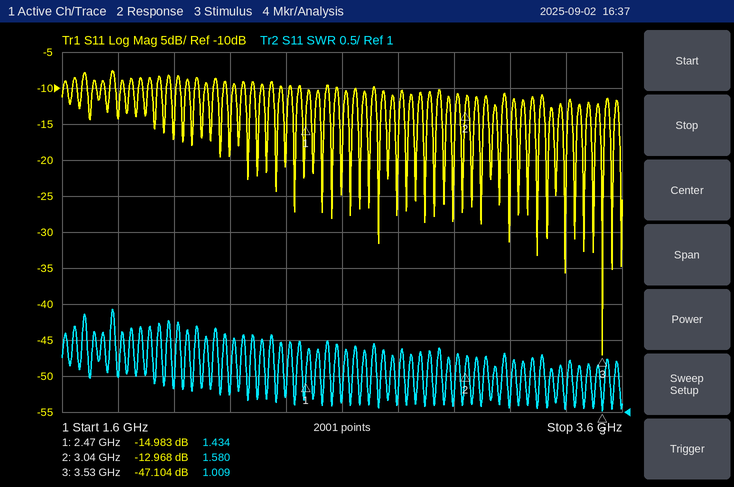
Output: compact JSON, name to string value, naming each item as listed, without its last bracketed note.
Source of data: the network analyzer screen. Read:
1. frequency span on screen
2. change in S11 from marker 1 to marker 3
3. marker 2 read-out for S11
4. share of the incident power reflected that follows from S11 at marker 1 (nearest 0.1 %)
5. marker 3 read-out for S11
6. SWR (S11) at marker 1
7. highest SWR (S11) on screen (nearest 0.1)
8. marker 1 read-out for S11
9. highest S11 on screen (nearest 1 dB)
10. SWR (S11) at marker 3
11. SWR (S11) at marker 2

{"frequency span on screen": "2 GHz", "change in S11 from marker 1 to marker 3": "-32.121 dB", "marker 2 read-out for S11": "-12.968 dB", "share of the incident power reflected that follows from S11 at marker 1": "3.2 %", "marker 3 read-out for S11": "-47.104 dB", "SWR (S11) at marker 1": "1.434", "highest SWR (S11) on screen": "2.4", "marker 1 read-out for S11": "-14.983 dB", "highest S11 on screen": "-8 dB", "SWR (S11) at marker 3": "1.009", "SWR (S11) at marker 2": "1.580"}
